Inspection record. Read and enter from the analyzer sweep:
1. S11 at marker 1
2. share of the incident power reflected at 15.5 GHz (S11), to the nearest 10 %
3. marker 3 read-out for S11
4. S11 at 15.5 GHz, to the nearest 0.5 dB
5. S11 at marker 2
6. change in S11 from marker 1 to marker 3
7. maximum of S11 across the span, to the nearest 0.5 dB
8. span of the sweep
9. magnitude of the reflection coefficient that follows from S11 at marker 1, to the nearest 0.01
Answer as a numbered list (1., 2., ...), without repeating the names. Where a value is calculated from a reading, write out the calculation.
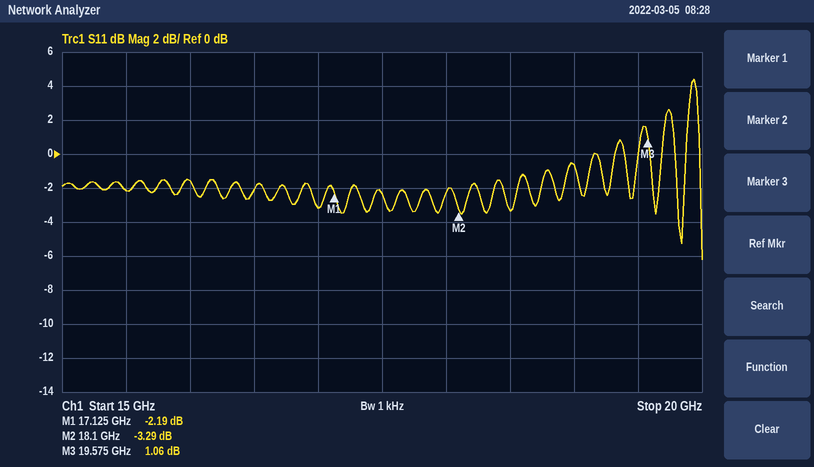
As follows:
1. -2.19 dB
2. 10^(-2/10) ≈ 63.1 %, so 60 % to the nearest 10 %
3. 1.06 dB
4. -2.0 dB
5. -3.29 dB
6. 1.06 − (-2.19) = 3.25 dB
7. 4.5 dB
8. 5 GHz
9. 10^(-2.19/20) ≈ 0.78
